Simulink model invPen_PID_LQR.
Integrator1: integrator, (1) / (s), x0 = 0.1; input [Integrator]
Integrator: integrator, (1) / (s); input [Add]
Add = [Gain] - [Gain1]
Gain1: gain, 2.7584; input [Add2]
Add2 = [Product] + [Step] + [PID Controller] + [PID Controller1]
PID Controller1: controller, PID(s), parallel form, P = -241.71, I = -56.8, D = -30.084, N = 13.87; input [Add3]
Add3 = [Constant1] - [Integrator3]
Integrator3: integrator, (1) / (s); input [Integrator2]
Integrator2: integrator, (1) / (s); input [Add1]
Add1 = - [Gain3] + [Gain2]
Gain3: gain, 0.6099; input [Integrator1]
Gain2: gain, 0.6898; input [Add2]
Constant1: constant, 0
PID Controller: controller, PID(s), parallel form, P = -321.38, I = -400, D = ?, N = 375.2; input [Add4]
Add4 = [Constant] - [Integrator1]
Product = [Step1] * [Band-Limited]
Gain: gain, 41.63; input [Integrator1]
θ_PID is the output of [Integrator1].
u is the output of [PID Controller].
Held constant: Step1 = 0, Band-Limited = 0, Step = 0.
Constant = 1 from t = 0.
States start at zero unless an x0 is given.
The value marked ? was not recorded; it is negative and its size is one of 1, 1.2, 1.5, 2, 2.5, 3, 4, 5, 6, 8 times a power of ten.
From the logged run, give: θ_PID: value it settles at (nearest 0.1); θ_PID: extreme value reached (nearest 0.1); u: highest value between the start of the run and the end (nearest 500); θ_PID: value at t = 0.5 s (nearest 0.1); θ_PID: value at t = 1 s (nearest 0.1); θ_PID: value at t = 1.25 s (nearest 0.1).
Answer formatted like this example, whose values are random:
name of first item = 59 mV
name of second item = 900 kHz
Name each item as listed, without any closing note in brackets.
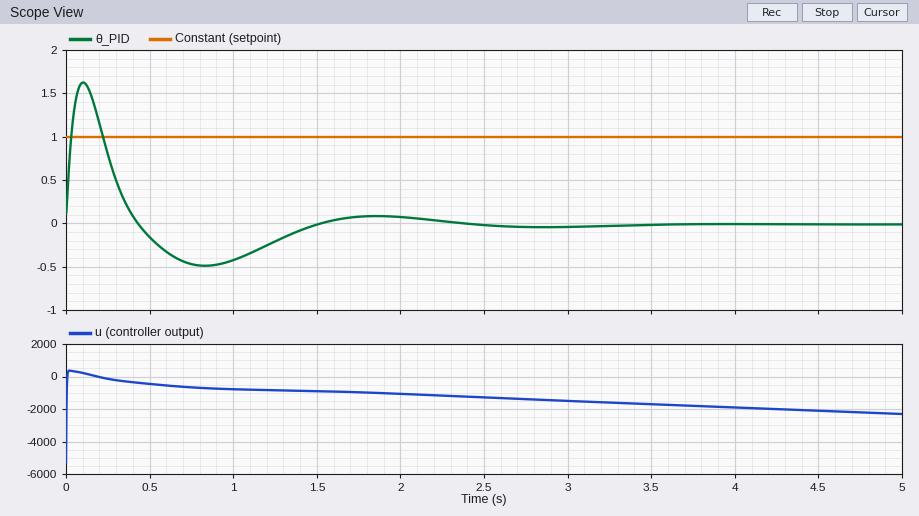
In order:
θ_PID: value it settles at = 0.0
θ_PID: extreme value reached = 1.6
u: highest value between the start of the run and the end = 500
θ_PID: value at t = 0.5 s = -0.2
θ_PID: value at t = 1 s = -0.4
θ_PID: value at t = 1.25 s = -0.2
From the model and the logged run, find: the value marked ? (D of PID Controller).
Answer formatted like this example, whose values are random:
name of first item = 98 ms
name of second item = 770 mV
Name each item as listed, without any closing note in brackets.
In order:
the value marked ? = -15
